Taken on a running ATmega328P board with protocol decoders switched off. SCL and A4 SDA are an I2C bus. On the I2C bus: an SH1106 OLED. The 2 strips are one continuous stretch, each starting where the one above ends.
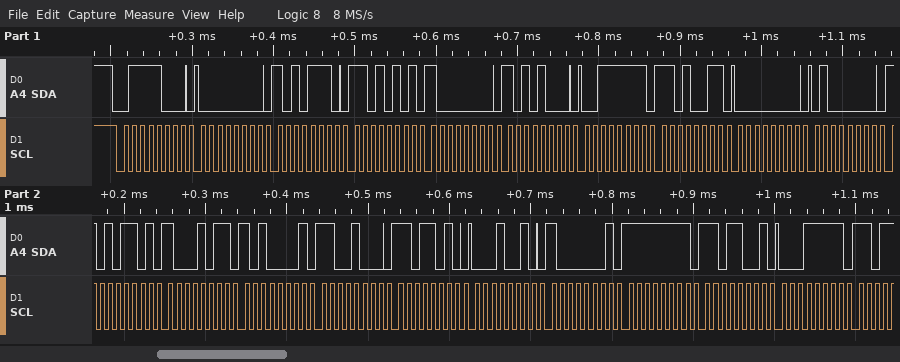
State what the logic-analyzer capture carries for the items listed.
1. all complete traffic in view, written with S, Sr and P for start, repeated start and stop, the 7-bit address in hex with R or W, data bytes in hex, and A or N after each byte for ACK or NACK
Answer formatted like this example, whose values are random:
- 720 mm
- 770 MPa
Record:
- S 3CW A 00 A AE A D5 A 80 A A8 A 3F A D3 A 00 A 40 A AD A 8B A A1 A C8 A DA A 12 A 81 A FF A D9 A 1F A
